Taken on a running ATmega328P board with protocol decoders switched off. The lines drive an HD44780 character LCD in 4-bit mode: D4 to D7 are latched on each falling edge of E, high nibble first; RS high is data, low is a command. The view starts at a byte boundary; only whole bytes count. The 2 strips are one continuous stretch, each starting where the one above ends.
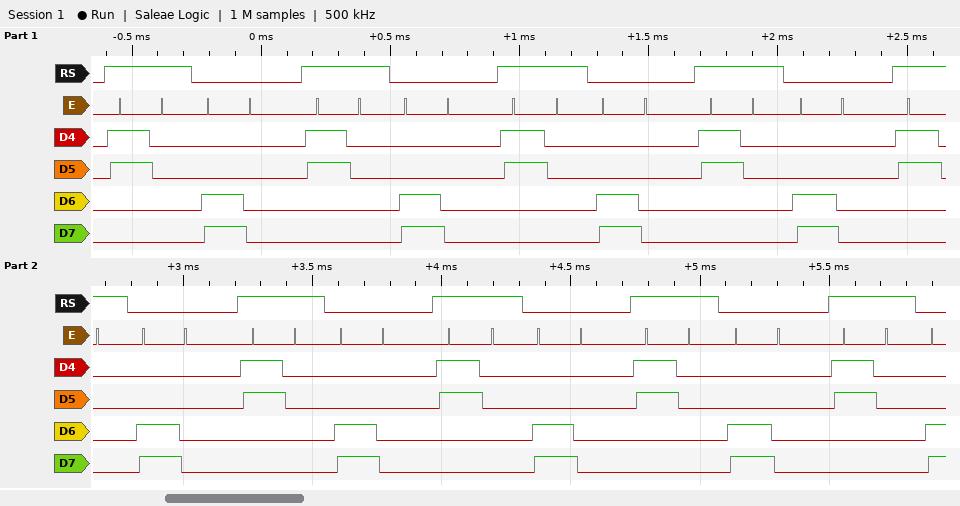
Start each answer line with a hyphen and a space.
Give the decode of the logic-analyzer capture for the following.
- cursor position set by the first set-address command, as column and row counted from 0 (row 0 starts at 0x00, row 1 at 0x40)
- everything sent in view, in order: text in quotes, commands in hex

- column 0, row 1
- "0" 0xC0 "0" 0xC0 "0" 0xC0 "0" 0xC0 "0" 0xC0 "0" 0xC0 "0" 0xC0 "0" 0xC0 "0"
